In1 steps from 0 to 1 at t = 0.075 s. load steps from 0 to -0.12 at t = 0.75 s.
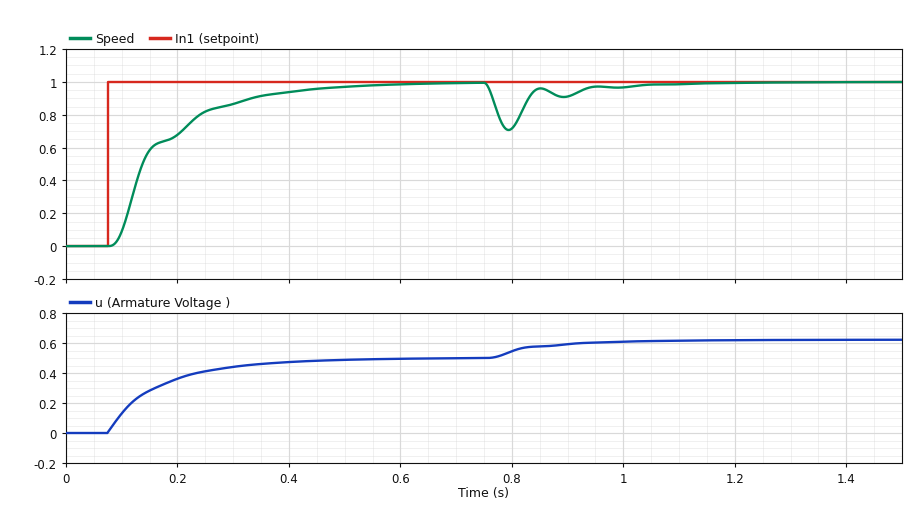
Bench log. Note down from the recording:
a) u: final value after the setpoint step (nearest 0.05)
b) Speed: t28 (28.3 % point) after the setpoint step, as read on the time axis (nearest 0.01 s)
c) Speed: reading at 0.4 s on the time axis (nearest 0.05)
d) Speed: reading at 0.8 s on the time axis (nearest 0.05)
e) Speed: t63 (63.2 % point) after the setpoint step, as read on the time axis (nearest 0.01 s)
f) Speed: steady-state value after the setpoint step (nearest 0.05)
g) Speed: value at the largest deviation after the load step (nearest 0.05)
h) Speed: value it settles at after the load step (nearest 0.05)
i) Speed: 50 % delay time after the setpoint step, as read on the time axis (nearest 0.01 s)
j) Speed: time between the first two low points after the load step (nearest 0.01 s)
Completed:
0.50
0.12 s
0.95
0.70
0.17 s
1.00
0.70
1.00
0.14 s
0.10 s
